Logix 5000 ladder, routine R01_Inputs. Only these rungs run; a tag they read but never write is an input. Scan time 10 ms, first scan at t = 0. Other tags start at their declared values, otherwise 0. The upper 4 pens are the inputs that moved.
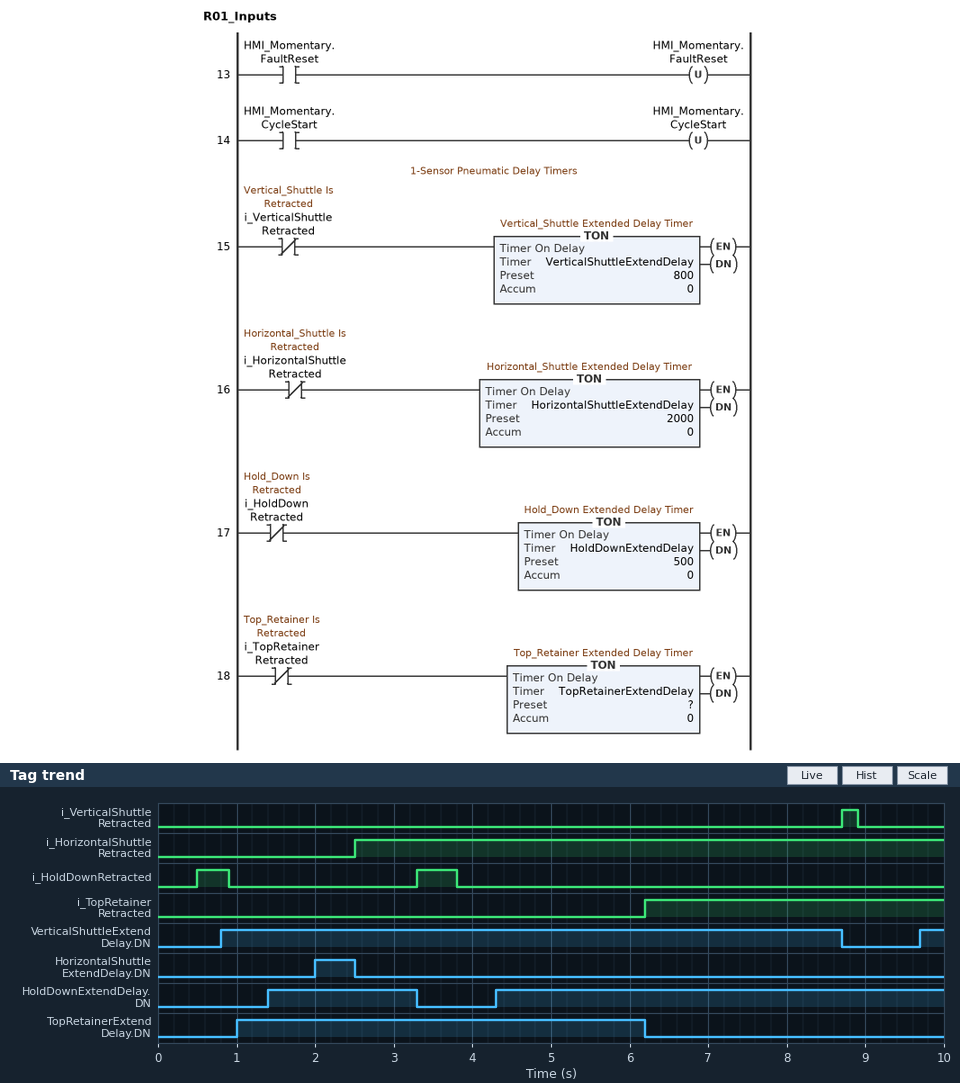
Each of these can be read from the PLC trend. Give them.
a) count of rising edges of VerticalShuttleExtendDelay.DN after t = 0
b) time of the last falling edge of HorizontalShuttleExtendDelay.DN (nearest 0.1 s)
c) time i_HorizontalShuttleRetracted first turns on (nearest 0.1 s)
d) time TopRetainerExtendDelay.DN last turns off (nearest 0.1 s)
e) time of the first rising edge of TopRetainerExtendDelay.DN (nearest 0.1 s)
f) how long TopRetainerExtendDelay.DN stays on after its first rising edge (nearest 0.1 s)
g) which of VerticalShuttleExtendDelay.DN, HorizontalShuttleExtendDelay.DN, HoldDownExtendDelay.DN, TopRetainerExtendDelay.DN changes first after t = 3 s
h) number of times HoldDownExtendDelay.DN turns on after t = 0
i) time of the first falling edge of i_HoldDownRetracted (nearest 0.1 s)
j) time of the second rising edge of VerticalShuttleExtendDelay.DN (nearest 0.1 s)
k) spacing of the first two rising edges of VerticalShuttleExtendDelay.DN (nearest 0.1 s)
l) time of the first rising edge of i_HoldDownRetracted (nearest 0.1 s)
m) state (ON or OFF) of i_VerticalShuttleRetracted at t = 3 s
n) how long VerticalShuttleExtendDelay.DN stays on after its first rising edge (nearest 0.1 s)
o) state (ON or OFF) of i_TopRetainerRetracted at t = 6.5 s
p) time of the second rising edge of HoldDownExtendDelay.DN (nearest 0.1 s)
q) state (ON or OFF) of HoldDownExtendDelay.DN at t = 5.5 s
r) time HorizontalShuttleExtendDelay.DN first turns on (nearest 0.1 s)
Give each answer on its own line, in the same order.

2
2.5 s
2.5 s
6.2 s
1.0 s
5.2 s
HoldDownExtendDelay.DN
2
0.9 s
9.7 s
8.9 s
0.5 s
OFF
7.9 s
ON
4.3 s
ON
2.0 s
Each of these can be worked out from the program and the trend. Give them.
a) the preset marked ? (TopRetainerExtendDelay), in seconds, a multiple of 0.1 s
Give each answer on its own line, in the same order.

1.0 s
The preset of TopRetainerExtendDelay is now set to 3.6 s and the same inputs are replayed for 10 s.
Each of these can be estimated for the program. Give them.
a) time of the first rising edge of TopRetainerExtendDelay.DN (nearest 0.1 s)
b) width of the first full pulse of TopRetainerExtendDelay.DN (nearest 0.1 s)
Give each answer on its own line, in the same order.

3.6 s
2.6 s
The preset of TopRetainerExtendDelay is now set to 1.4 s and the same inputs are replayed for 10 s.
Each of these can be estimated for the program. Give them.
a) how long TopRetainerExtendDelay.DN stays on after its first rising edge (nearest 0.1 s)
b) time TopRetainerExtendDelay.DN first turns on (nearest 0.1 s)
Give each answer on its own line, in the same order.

4.8 s
1.4 s
